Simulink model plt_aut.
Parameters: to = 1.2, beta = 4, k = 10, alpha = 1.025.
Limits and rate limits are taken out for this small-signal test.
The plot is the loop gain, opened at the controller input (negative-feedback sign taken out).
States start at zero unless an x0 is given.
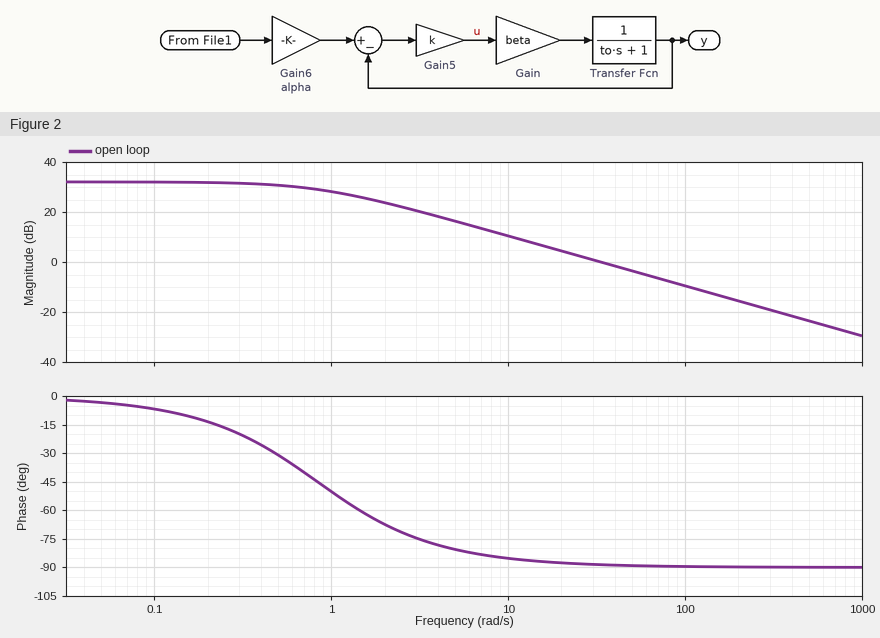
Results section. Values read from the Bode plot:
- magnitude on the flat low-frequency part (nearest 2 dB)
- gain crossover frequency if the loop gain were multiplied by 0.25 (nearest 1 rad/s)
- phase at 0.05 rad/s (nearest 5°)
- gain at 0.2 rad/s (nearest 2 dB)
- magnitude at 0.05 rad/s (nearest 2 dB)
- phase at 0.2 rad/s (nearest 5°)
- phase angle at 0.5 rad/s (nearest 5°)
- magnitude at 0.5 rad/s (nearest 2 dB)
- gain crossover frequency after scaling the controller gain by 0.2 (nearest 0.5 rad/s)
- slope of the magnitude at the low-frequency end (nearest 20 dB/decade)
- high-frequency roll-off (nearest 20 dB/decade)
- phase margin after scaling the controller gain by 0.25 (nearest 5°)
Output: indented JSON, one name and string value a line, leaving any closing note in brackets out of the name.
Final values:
{
  "magnitude on the flat low-frequency part": "32 dB",
  "gain crossover frequency if the loop gain were multiplied by 0.25": "8 rad/s",
  "phase at 0.05 rad/s": "-5°",
  "gain at 0.2 rad/s": "32 dB",
  "magnitude at 0.05 rad/s": "32 dB",
  "phase at 0.2 rad/s": "-15°",
  "phase angle at 0.5 rad/s": "-30°",
  "magnitude at 0.5 rad/s": "30 dB",
  "gain crossover frequency after scaling the controller gain by 0.2": "6.5 rad/s",
  "slope of the magnitude at the low-frequency end": "0 dB/decade",
  "high-frequency roll-off": "-20 dB/decade",
  "phase margin after scaling the controller gain by 0.25": "95°"
}
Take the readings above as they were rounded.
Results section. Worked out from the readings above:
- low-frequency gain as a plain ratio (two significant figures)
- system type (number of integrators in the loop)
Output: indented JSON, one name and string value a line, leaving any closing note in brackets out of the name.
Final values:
{
  "low-frequency gain as a plain ratio": "40",
  "system type": "0"
}
